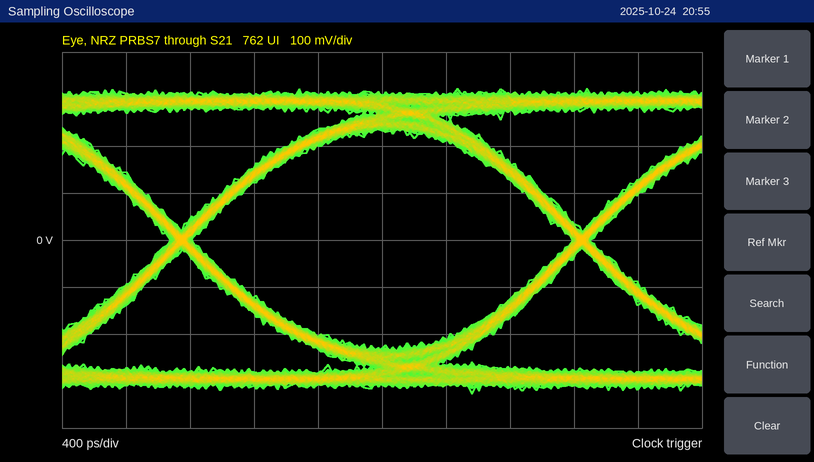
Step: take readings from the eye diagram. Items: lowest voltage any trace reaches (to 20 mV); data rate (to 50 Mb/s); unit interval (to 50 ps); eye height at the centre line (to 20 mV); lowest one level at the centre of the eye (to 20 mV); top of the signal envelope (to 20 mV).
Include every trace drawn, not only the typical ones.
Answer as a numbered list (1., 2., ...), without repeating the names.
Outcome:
1. -320 mV
2. 400 Mb/s
3. 2.50 ns
4. 460 mV
5. 240 mV
6. 320 mV
